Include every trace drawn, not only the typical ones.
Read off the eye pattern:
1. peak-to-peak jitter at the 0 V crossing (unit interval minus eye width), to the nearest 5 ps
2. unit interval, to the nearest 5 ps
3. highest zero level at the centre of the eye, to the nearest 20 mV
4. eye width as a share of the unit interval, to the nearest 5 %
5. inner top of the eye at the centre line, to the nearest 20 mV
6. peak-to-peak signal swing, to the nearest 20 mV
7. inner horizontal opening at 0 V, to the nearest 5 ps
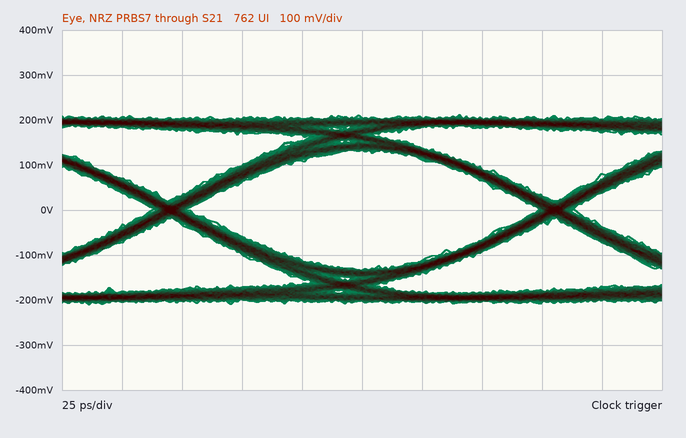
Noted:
15 ps
160 ps
-140 mV
90 %
140 mV
420 mV
145 ps
